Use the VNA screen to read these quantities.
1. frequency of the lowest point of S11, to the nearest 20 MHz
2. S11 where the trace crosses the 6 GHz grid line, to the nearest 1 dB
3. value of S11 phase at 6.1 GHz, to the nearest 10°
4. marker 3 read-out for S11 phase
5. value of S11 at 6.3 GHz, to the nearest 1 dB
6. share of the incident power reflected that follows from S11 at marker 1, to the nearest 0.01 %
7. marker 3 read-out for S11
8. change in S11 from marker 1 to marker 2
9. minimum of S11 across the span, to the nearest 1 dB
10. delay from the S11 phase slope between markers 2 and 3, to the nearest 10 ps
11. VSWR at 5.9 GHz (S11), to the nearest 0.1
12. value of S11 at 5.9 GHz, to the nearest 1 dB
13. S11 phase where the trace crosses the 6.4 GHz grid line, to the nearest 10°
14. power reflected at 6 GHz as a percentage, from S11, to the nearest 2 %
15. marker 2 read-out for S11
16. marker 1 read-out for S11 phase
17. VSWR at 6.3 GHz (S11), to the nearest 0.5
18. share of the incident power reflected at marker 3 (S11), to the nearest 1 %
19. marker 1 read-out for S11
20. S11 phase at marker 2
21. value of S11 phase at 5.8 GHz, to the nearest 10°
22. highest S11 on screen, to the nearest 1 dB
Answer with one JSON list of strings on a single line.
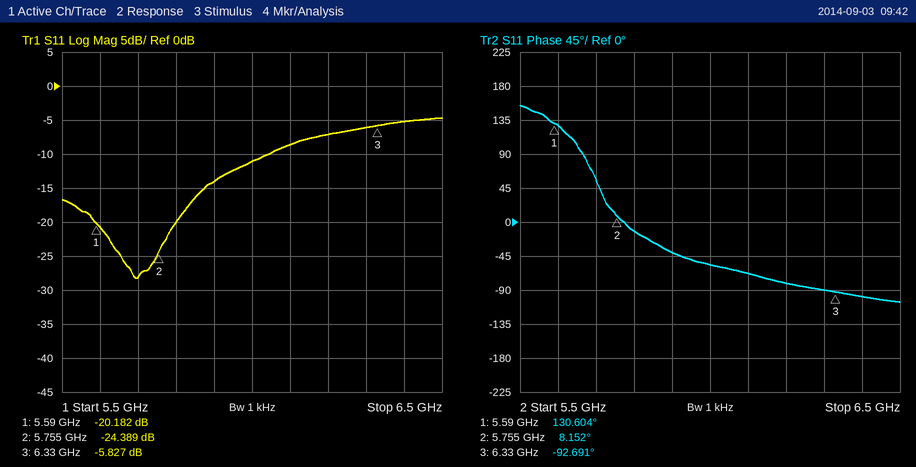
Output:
["5.70 GHz", "-11 dB", "-70°", "-92.691°", "-6 dB", "0.96 %", "-5.827 dB", "-4.207 dB", "-28 dB", "490 ps", "1.5", "-14 dB", "-100°", "8 %", "-24.389 dB", "130.604°", "3.0", "26 %", "-20.182 dB", "8.152°", "-10°", "-5 dB"]
